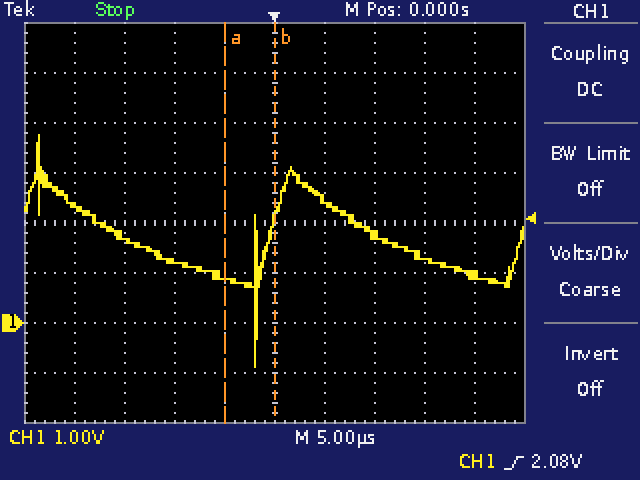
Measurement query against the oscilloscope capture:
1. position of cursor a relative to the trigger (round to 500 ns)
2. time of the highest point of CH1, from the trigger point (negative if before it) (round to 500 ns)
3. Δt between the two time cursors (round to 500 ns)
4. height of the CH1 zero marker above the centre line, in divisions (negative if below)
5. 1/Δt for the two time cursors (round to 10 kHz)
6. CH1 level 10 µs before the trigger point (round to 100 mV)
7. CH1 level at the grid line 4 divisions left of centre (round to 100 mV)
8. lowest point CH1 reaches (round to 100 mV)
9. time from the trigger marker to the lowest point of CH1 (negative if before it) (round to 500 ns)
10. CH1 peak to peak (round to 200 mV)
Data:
-5.0 µs
-23.5 µs
5.0 µs
-2.0 div
200 kHz
1.2 V
2.3 V
-900 mV
-2.0 µs
4.6 V
